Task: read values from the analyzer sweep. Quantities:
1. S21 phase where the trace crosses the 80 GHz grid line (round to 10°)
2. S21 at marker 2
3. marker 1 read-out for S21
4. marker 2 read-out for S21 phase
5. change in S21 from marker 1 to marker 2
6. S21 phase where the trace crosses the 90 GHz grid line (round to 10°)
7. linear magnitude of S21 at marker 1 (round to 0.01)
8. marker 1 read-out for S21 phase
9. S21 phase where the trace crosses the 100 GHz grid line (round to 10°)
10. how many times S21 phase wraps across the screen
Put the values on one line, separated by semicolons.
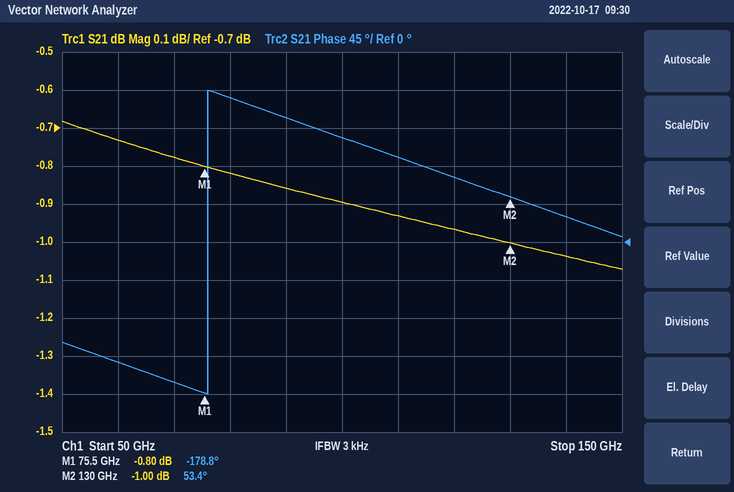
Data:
170°; -1.00 dB; -0.80 dB; 53.4°; -0.20 dB; 150°; 0.91; -178.8°; 120°; 1
